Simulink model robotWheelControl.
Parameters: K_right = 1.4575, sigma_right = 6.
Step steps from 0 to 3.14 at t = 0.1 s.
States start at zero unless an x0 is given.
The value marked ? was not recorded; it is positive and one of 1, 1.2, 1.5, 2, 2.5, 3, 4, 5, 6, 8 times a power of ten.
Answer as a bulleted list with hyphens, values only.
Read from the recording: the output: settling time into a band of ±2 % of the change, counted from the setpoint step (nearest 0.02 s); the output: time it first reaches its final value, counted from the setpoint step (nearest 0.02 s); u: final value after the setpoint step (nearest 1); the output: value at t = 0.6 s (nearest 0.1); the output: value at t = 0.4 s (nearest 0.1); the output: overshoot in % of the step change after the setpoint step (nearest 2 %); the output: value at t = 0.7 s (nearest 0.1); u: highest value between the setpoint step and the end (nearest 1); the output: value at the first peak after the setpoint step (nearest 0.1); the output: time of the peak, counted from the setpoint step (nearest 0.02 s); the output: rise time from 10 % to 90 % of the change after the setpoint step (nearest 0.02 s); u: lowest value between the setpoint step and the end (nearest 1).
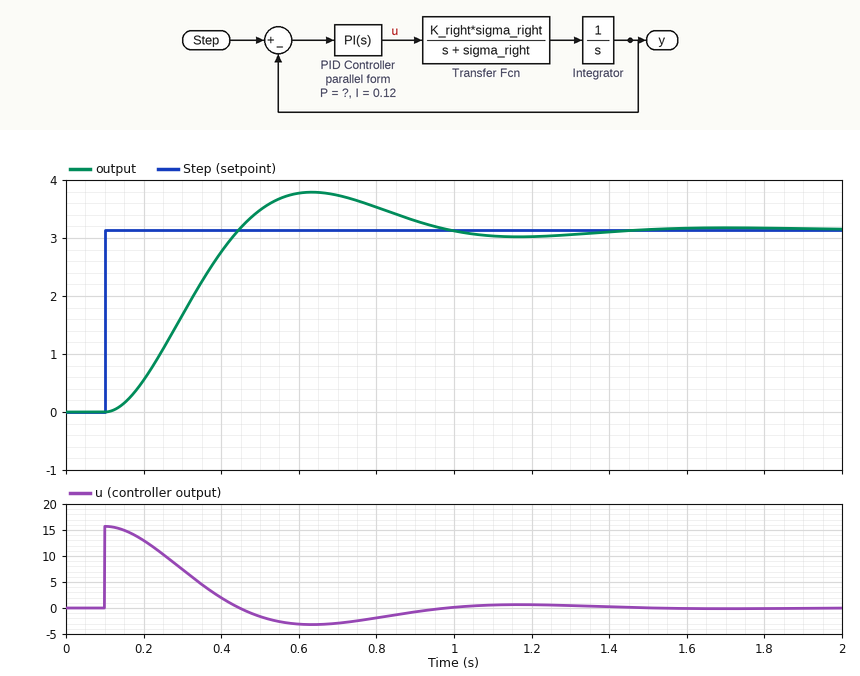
- 1.26 s
- 0.34 s
- 0
- 3.8
- 2.8
- 20 %
- 3.7
- 16
- 3.8
- 0.54 s
- 0.24 s
- -3
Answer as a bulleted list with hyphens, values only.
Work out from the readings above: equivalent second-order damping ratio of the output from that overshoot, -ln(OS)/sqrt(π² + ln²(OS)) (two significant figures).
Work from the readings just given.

- 0.46
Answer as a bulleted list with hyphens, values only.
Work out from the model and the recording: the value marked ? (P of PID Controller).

- 5
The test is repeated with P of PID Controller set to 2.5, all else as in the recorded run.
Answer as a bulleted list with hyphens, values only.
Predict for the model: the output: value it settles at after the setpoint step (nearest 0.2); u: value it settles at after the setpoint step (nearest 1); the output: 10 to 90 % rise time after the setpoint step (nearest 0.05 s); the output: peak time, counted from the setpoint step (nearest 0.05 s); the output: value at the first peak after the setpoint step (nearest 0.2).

- 3.2
- 0
- 0.40 s
- 0.90 s
- 3.4
